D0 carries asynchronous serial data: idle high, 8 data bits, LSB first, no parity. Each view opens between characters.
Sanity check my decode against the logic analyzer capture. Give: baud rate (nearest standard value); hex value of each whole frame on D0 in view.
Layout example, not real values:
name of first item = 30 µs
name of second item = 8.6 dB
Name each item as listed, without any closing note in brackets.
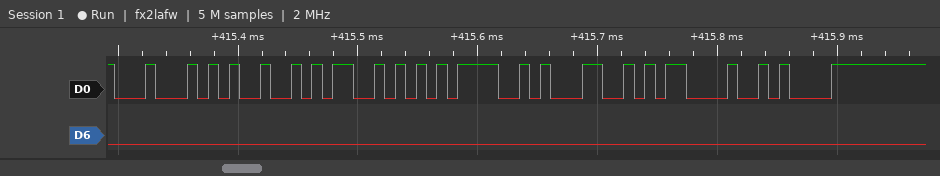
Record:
baud rate = 115200 baud
hex value of each whole frame on D0 in view = 44, 49, 53, 3D, 31, 0D, 0A
